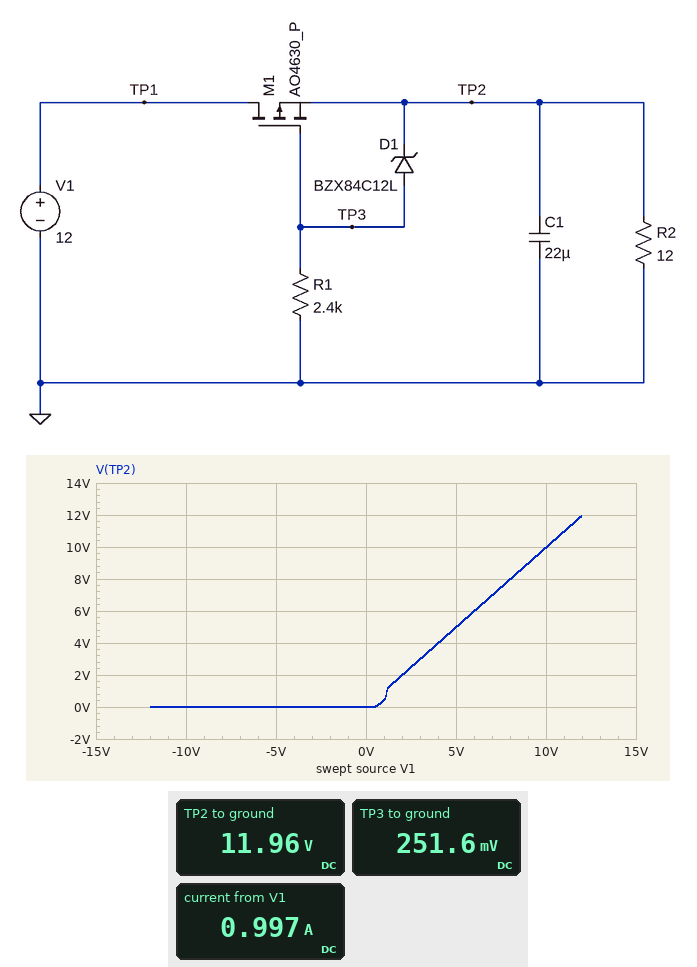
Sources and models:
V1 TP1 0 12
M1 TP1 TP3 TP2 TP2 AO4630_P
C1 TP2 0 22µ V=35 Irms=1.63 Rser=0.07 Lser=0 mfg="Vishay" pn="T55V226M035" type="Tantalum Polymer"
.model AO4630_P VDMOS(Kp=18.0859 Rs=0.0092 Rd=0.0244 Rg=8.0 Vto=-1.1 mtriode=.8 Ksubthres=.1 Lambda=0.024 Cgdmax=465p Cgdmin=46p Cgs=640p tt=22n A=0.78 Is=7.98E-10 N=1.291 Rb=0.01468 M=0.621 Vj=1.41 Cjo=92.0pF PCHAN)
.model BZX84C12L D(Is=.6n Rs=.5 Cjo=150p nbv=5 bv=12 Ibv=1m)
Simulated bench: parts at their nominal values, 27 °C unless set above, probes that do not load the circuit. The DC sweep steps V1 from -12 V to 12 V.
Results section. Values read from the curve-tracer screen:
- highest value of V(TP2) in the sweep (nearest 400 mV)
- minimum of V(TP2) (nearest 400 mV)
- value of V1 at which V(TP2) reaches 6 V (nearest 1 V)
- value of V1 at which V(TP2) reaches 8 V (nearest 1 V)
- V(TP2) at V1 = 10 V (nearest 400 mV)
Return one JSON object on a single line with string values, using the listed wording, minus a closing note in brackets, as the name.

{"highest value of V(TP2) in the sweep": "12.0 V", "minimum of V(TP2)": "0 V", "value of V1 at which V(TP2) reaches 6 V": "6 V", "value of V1 at which V(TP2) reaches 8 V": "8 V", "V(TP2) at V1 = 10 V": "10.0 V"}
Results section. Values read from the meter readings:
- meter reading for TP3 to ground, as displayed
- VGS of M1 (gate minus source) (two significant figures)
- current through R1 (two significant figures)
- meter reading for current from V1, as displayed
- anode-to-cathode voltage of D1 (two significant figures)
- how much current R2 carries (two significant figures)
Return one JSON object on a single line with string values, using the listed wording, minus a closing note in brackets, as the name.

{"meter reading for TP3 to ground, as displayed": "251.6 mV", "VGS of M1 (gate minus source)": "-12 V", "current through R1": "100 µA", "meter reading for current from V1, as displayed": "0.997 A", "anode-to-cathode voltage of D1": "-12 V", "how much current R2 carries": "1.0 A"}
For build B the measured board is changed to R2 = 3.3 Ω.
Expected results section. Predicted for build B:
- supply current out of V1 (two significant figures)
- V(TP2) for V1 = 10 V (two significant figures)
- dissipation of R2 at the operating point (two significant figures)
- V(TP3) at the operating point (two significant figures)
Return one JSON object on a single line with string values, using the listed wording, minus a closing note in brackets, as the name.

{"supply current out of V1": "3.6 A", "V(TP2) for V1 = 10 V": "9.9 V", "dissipation of R2 at the operating point": "43 W", "V(TP3) at the operating point": "190 mV"}
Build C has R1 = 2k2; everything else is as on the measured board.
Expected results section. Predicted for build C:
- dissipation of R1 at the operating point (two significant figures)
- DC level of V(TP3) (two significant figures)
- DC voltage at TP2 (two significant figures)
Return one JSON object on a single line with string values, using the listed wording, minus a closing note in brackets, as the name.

{"dissipation of R1 at the operating point": "27 µW", "DC level of V(TP3)": "240 mV", "DC voltage at TP2": "12 V"}
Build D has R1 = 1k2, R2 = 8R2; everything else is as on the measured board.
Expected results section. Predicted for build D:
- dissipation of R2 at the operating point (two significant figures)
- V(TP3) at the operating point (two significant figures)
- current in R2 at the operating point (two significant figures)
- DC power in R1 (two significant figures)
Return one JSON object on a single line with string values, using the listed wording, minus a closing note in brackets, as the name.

{"dissipation of R2 at the operating point": "17 W", "V(TP3) at the operating point": "180 mV", "current in R2 at the operating point": "1.5 A", "DC power in R1": "28 µW"}
